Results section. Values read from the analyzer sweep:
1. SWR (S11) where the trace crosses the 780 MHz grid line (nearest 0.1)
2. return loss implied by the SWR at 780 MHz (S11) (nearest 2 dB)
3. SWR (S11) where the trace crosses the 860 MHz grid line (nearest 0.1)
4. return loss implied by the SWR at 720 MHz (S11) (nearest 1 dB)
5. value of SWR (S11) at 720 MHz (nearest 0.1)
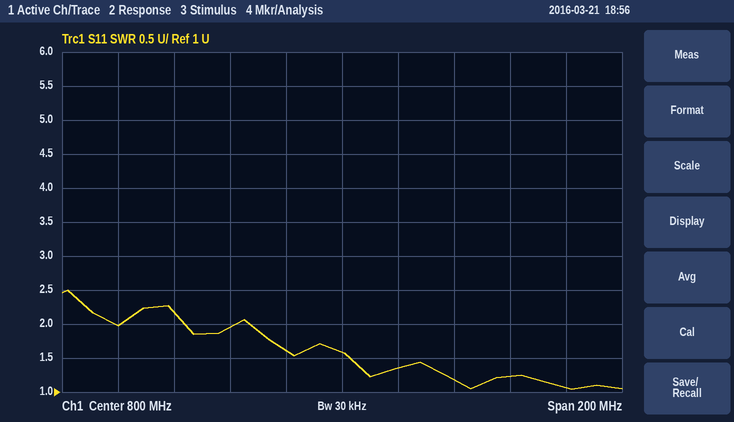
1.6
12 dB
1.2
10 dB
2.0
